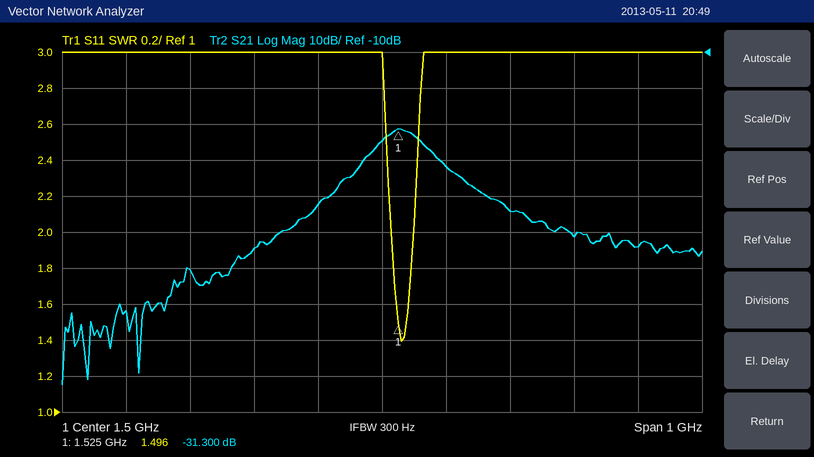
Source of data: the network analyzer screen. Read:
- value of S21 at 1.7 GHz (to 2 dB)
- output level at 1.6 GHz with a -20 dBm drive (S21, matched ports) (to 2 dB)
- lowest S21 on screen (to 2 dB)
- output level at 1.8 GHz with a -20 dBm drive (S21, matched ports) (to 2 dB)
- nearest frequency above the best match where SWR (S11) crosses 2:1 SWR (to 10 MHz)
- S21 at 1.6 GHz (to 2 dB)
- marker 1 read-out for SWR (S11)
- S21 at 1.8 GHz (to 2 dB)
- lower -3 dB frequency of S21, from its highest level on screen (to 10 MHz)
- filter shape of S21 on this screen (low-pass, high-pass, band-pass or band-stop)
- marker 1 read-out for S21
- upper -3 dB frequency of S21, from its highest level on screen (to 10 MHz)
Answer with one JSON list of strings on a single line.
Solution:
["-54 dB", "-62 dBm", "-102 dB", "-82 dBm", "1.55 GHz", "-42 dB", "1.496", "-62 dB", "1.50 GHz", "band-pass", "-31.300 dB", "1.56 GHz"]
